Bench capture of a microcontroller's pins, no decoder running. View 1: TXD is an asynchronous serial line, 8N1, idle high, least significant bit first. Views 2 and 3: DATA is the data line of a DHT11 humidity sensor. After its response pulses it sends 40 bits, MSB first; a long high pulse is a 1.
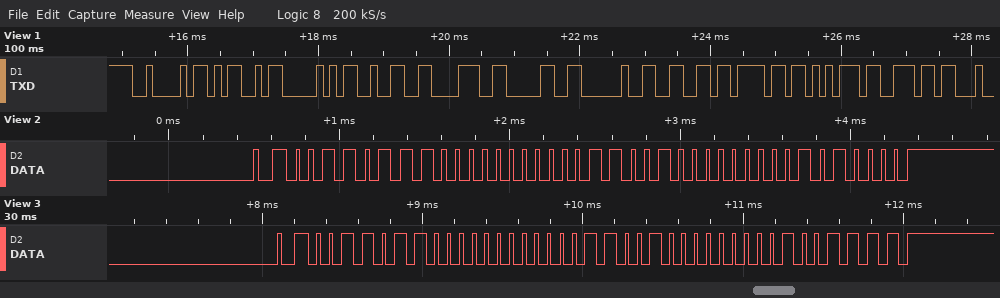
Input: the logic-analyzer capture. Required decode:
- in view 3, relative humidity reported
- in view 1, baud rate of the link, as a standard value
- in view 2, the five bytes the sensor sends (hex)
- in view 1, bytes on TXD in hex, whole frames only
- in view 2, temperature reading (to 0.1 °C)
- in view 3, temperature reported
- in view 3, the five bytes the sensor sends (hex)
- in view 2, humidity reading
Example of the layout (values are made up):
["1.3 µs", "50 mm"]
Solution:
["54 %", "9600 baud", "37 00 19 00 50", "0x42 0x4D 0x50 0x32 0x38 0x30 0x20 0x66 0x6F 0x75 0x6E", "25.0 °C", "25.0 °C", "36 00 19 00 4F", "55 %"]
